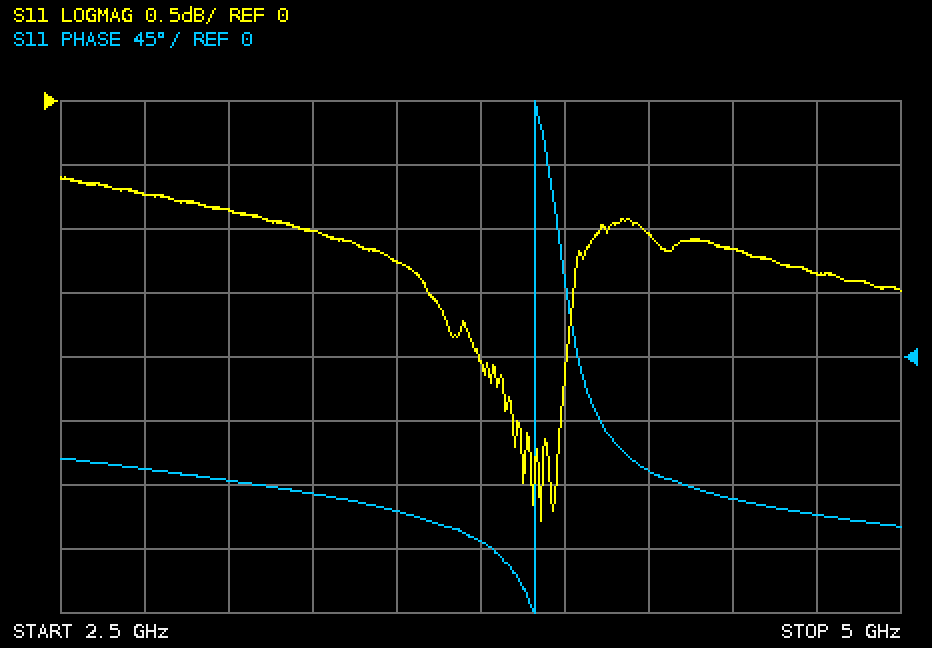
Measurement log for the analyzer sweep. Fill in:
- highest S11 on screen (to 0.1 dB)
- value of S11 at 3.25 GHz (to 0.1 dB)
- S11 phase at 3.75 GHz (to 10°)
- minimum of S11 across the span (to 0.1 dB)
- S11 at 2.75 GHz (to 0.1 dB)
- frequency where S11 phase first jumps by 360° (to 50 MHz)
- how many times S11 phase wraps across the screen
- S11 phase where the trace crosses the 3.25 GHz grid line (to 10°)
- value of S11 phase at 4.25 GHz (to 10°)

-0.6 dB
-1.0 dB
-130°
-3.3 dB
-0.7 dB
3.90 GHz
1
-100°
-80°
